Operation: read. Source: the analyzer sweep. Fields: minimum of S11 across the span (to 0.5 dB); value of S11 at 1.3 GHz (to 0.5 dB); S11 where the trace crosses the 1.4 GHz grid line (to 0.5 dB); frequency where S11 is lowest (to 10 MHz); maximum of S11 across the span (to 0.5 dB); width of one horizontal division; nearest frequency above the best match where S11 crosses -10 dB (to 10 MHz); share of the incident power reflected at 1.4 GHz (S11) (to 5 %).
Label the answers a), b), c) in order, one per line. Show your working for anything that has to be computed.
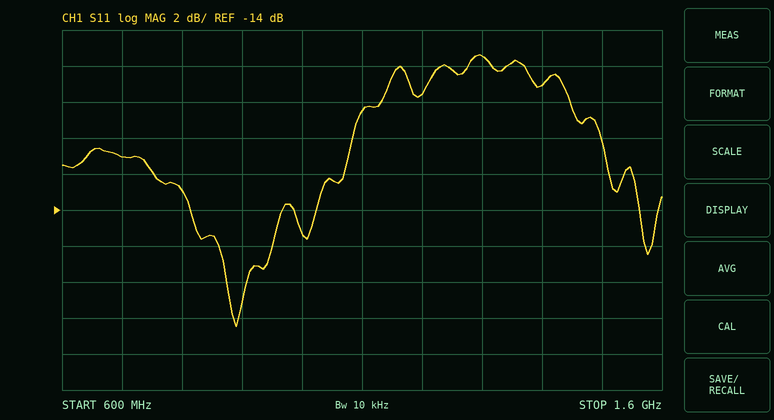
a) -20.5 dB
b) -5.5 dB
c) -7.0 dB
d) 890 MHz
e) -5.5 dB
f) 100 MHz
g) 1.08 GHz
h) 10^(-7/10) ≈ 20 %
